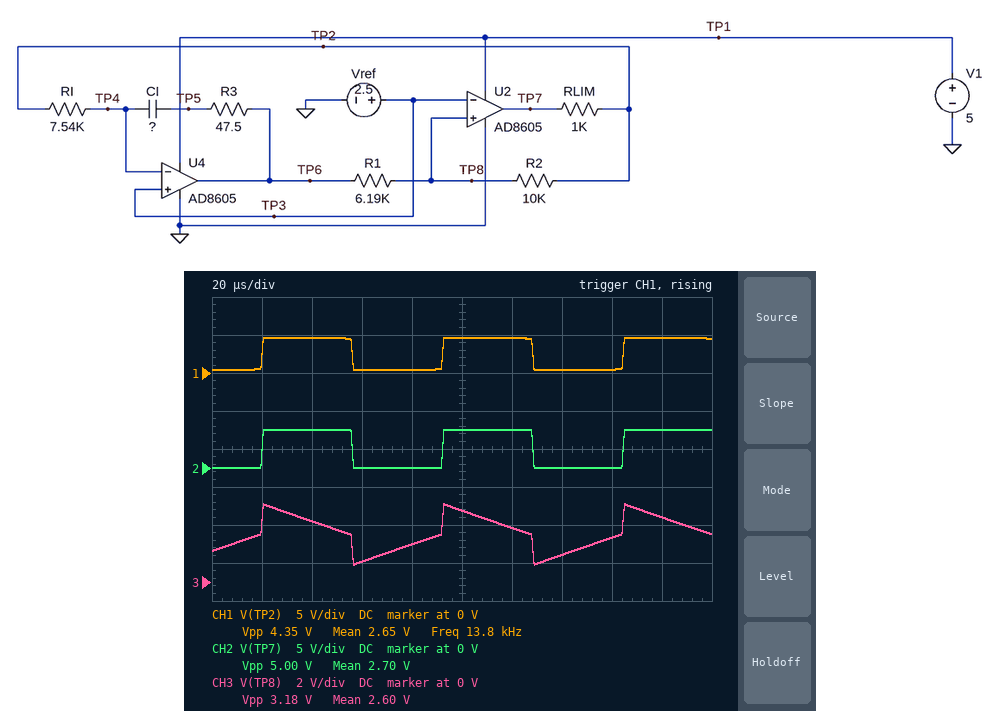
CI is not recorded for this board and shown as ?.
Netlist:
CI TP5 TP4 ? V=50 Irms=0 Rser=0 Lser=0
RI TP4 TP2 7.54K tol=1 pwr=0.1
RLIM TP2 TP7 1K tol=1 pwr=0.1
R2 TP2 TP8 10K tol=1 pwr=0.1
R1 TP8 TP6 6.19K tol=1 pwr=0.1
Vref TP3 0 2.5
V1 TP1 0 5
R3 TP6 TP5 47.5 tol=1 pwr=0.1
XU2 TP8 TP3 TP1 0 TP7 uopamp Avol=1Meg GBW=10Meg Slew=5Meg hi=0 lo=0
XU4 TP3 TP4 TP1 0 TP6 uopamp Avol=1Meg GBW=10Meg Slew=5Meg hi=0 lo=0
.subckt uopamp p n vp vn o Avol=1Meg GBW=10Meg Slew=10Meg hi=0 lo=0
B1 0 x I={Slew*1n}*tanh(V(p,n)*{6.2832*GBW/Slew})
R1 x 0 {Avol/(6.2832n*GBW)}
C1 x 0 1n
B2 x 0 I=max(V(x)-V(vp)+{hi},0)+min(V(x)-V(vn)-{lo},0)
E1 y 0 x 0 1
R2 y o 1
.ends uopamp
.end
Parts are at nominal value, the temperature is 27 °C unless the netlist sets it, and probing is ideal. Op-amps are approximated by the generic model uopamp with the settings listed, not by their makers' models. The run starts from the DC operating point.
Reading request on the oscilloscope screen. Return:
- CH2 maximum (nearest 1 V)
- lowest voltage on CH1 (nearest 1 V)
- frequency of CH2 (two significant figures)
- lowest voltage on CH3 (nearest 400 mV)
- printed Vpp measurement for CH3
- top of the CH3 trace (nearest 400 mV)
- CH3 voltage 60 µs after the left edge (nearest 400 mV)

5 V
0 V
14 kHz
800 mV
3.18 V
4.0 V
1.2 V
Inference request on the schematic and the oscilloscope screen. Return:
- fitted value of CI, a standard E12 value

3.9 nF
